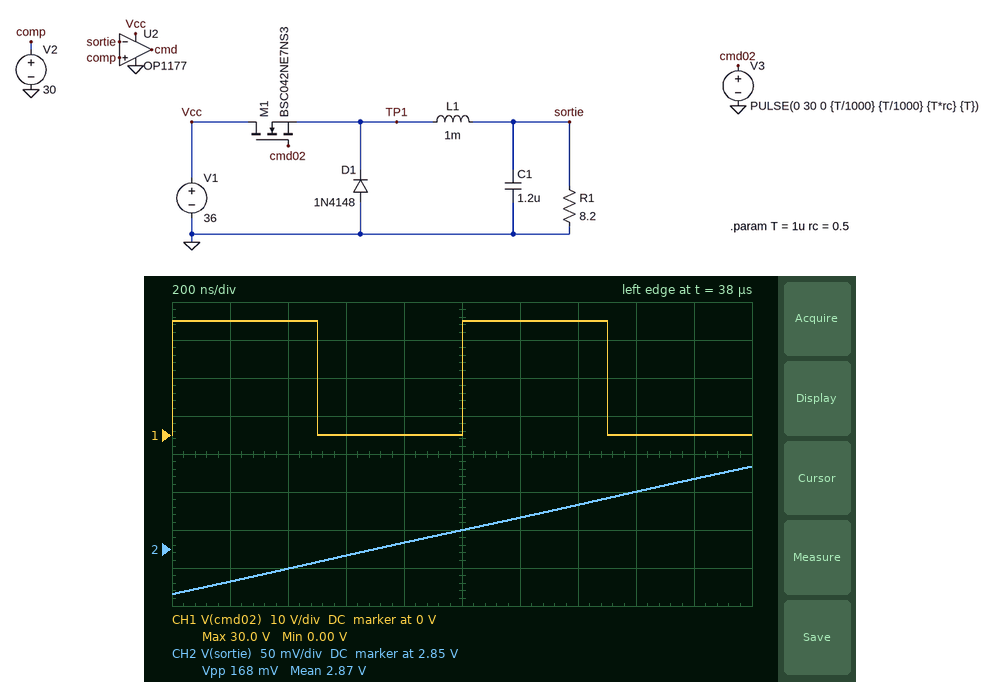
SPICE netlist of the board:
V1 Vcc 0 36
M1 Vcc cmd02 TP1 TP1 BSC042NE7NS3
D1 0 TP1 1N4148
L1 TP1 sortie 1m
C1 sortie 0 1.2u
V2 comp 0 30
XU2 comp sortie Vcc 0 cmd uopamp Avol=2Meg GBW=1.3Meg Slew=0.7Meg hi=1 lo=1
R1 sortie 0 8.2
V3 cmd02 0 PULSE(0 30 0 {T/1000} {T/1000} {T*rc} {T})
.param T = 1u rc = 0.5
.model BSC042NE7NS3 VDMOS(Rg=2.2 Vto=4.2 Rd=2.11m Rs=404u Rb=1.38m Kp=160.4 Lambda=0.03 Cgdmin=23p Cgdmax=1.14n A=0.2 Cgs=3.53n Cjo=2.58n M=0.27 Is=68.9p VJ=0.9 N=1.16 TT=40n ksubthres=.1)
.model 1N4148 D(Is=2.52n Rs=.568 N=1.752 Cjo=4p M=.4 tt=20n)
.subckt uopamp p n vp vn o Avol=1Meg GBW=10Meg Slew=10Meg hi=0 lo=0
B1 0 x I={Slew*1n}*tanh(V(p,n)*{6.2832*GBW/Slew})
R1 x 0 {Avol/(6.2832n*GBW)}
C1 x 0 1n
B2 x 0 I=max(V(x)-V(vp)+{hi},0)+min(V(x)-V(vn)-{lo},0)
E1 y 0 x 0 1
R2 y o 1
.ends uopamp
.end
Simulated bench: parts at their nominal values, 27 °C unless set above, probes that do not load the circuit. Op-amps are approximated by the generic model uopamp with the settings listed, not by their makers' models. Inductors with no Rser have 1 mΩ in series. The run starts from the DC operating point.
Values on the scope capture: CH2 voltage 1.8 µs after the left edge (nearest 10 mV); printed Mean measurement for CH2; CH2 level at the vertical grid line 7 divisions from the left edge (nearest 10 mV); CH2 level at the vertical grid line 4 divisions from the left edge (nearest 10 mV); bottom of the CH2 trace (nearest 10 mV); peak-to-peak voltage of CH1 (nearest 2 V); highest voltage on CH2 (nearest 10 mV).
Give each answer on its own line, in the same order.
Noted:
2.94 V
2.87 V
2.91 V
2.86 V
2.79 V
30 V
2.96 V
